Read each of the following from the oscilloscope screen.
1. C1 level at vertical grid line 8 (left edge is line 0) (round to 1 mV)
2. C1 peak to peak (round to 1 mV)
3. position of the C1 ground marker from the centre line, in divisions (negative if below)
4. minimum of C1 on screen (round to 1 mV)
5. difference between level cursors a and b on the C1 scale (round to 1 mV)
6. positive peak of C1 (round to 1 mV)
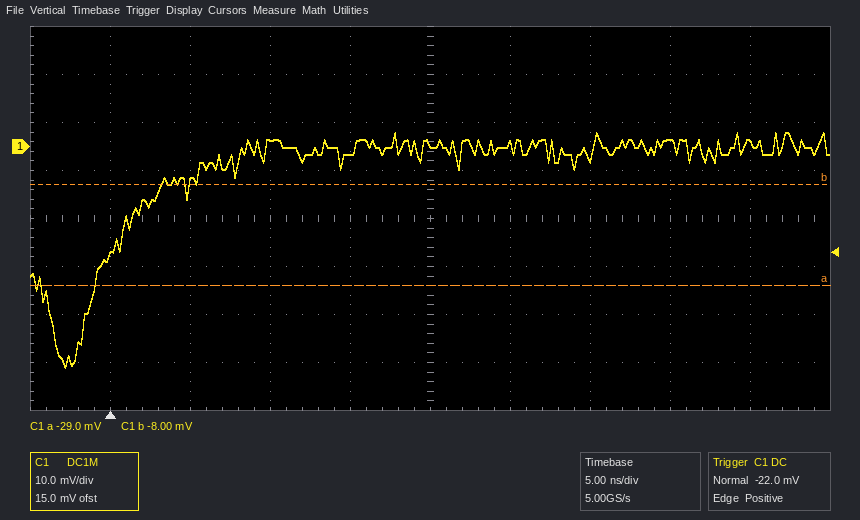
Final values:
1 mV
49 mV
+1.5 div
-46 mV
21 mV
3 mV
